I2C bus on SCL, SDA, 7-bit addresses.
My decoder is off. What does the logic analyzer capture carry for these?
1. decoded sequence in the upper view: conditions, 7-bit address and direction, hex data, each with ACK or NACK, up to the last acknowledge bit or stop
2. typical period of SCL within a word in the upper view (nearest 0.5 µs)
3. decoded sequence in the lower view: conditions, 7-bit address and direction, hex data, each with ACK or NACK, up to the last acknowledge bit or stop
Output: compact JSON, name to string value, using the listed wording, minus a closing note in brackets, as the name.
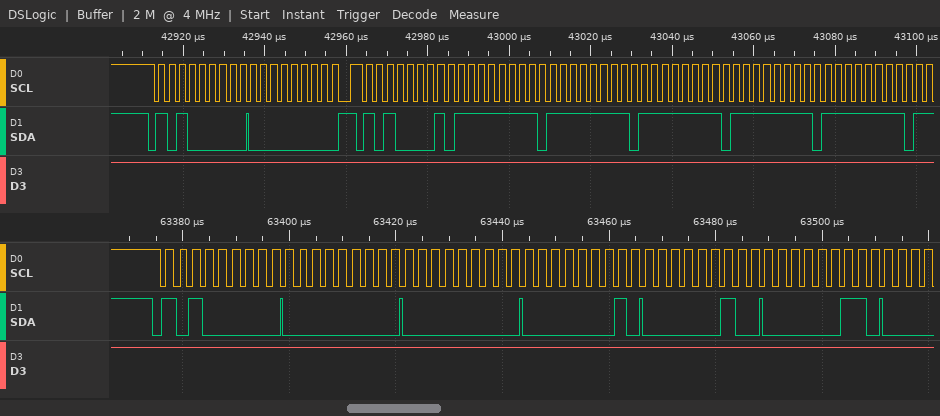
{"decoded sequence in the upper view: conditions, 7-bit address and direction, hex data, each with ACK or NACK, up to the last acknowledge bit or stop": "start, address 50 write ACK, 00 ACK, repeated start, address 50 read ACK, FF ACK, FF ACK, FF ACK, FF ACK, FF ACK", "typical period of SCL within a word in the upper view": "2.5 µs", "decoded sequence in the lower view: conditions, 7-bit address and direction, hex data, each with ACK or NACK, up to the last acknowledge bit or stop": "start, address 50 write ACK, 00 ACK, 00 ACK, 01 ACK, 02 ACK, 03 ACK"}
